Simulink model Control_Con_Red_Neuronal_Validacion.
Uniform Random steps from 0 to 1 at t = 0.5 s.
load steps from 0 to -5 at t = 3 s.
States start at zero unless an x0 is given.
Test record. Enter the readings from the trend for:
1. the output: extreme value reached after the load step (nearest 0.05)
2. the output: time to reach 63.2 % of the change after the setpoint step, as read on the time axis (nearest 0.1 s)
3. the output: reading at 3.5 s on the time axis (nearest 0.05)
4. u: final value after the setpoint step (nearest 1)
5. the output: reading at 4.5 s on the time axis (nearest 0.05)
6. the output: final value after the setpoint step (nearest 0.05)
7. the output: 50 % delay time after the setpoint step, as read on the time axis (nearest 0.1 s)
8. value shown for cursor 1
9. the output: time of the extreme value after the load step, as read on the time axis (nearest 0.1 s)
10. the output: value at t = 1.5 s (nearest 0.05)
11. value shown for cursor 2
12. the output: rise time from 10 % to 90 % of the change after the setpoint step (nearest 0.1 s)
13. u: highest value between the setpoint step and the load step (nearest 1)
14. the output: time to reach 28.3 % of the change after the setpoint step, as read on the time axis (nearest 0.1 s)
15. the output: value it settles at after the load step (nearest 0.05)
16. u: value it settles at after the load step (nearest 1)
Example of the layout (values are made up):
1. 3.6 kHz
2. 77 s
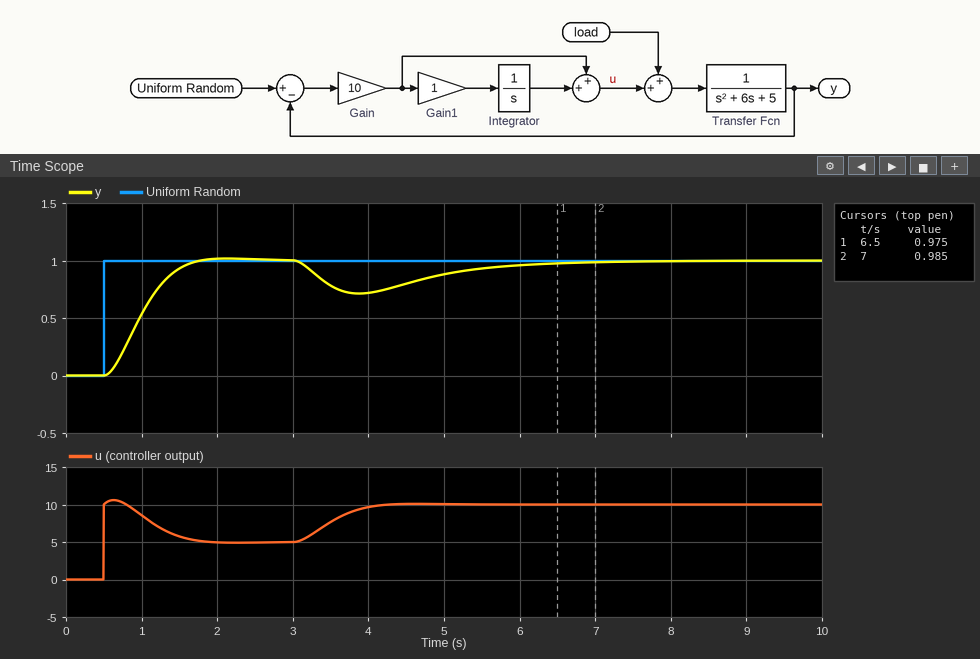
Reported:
1. 0.70
2. 1.1 s
3. 0.80
4. 5
5. 0.80
6. 1.00
7. 1.0 s
8. 0.975
9. 3.9 s
10. 0.95
11. 0.985
12. 0.8 s
13. 11
14. 0.8 s
15. 1.00
16. 10
